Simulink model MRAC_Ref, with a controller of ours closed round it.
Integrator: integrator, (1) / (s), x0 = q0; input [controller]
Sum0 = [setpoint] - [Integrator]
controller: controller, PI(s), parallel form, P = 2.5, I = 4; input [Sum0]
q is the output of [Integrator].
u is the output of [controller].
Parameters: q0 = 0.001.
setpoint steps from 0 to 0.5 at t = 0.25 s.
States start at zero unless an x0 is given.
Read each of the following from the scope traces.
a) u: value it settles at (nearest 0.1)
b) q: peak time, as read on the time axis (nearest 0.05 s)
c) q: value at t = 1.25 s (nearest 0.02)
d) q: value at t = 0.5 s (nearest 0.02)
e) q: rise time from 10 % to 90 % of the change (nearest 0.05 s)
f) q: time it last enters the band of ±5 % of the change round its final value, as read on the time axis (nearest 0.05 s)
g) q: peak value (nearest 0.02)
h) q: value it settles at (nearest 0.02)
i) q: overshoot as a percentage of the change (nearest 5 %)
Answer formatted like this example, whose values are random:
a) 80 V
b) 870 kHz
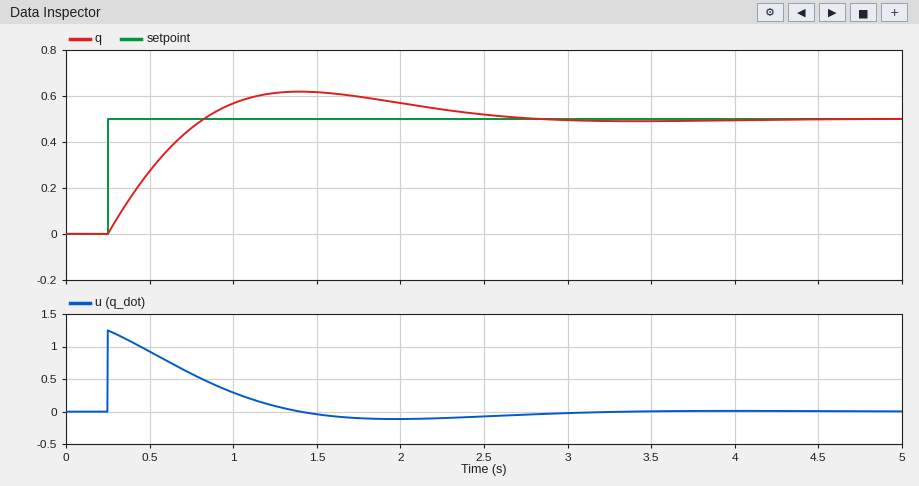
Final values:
a) 0.0
b) 1.40 s
c) 0.62
d) 0.28
e) 0.45 s
f) 2.45 s
g) 0.62
h) 0.50
i) 25 %
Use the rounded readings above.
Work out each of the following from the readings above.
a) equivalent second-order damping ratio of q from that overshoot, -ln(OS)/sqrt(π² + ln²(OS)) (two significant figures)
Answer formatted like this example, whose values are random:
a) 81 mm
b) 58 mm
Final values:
a) 0.40
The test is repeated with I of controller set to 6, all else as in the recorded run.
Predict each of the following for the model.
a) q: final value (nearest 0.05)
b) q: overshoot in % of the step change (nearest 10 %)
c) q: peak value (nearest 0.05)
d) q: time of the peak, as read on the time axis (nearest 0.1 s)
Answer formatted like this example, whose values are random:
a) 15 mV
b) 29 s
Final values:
a) 0.50
b) 30 %
c) 0.65
d) 1.2 s
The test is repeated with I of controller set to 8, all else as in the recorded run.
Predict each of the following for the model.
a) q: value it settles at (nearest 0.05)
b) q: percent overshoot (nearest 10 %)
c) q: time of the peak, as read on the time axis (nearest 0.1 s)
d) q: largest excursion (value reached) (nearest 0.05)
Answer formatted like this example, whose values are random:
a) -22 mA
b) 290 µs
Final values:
a) 0.50
b) 30 %
c) 1.1 s
d) 0.65
